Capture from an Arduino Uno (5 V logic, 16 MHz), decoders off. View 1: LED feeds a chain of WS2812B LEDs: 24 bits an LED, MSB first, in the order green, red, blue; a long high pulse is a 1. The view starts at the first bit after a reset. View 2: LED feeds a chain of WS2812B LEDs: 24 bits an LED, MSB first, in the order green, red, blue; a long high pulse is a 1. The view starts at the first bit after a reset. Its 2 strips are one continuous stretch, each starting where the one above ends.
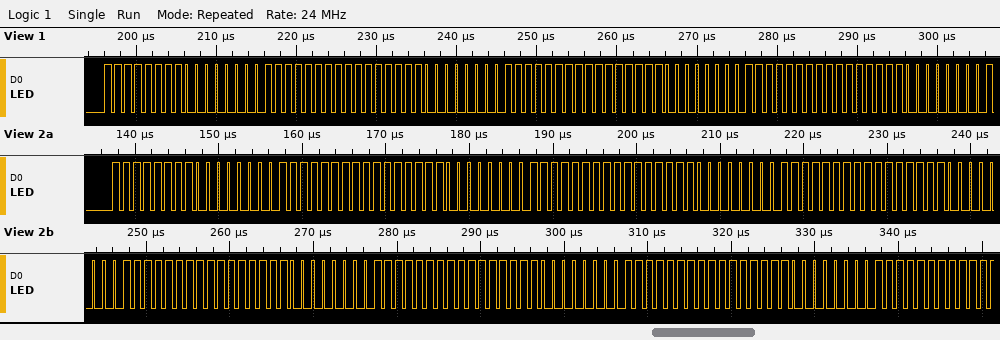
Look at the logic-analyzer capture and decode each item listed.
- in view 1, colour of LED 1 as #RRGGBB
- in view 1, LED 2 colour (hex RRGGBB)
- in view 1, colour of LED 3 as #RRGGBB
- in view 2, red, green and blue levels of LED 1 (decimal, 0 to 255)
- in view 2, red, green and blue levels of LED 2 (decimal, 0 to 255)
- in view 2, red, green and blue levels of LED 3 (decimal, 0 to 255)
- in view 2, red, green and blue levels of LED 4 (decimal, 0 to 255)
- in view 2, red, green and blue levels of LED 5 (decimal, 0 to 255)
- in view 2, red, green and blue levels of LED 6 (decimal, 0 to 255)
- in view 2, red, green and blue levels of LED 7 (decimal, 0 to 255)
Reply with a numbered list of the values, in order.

1. #00FFFF
2. #00FFFF
3. #00FFFF
4. 0, 255, 255
5. 0, 255, 255
6. 0, 255, 255
7. 0, 255, 255
8. 0, 255, 255
9. 0, 255, 255
10. 0, 255, 255
